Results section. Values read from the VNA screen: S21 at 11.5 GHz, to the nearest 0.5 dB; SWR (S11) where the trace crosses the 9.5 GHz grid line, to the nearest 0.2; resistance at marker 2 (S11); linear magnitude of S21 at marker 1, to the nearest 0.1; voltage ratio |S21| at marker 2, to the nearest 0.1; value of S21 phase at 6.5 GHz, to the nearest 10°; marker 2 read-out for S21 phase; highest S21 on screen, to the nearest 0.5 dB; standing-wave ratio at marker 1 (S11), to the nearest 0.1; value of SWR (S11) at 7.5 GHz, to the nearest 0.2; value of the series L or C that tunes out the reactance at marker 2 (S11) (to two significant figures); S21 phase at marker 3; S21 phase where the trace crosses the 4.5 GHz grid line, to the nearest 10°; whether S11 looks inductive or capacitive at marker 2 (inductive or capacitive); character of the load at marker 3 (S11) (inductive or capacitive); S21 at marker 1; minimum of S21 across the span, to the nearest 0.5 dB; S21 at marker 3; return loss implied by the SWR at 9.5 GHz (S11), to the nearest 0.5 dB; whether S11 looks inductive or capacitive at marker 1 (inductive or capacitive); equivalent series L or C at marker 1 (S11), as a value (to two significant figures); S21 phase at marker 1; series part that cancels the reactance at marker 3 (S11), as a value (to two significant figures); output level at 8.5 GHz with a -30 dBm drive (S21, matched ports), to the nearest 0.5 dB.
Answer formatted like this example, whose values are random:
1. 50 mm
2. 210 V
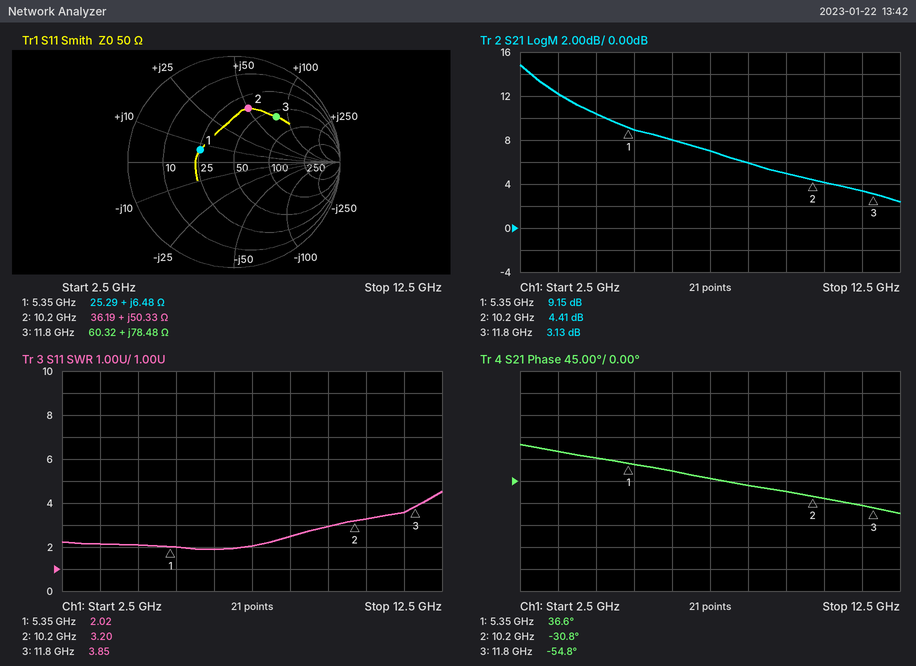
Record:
1. 3.5 dB
2. 3.0
3. 36.19 Ω
4. 2.9
5. 1.7
6. 20°
7. -30.8°
8. 15.0 dB
9. 2.0
10. 2.0
11. 310 fF
12. -54.8°
13. 50°
14. inductive
15. inductive
16. 9.15 dB
17. 2.5 dB
18. 3.13 dB
19. 6.0 dB
20. inductive
21. 190 pH
22. 36.6°
23. 170 fF
24. -24.0 dBm
